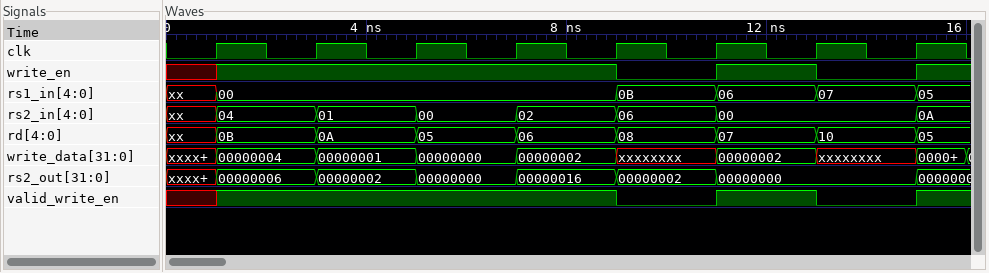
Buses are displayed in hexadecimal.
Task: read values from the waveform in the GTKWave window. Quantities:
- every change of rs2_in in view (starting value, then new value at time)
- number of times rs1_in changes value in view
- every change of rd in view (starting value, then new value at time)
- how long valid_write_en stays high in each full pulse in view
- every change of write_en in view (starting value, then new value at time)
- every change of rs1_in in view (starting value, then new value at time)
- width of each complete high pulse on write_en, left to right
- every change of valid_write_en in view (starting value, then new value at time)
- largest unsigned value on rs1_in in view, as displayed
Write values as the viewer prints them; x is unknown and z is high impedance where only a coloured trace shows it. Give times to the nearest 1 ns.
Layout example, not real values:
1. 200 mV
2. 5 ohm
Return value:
1. xx, 04 at 1 ns, 01 at 3 ns, 00 at 5 ns, 02 at 7 ns, 06 at 9 ns, 00 at 11 ns, 0A at 15 ns
2. 5
3. xx, 0B at 1 ns, 0A at 3 ns, 05 at 5 ns, 06 at 7 ns, 08 at 9 ns, 07 at 11 ns, 10 at 13 ns, 05 at 15 ns
4. 2 ns
5. x, 1 at 1 ns, 0 at 9 ns, 1 at 11 ns, 0 at 13 ns, 1 at 15 ns
6. xx, 00 at 1 ns, 0B at 9 ns, 06 at 11 ns, 07 at 13 ns, 05 at 15 ns
7. 2 ns
8. x, 1 at 1 ns, 0 at 9 ns, 1 at 11 ns, 0 at 13 ns, 1 at 15 ns
9. 0B
